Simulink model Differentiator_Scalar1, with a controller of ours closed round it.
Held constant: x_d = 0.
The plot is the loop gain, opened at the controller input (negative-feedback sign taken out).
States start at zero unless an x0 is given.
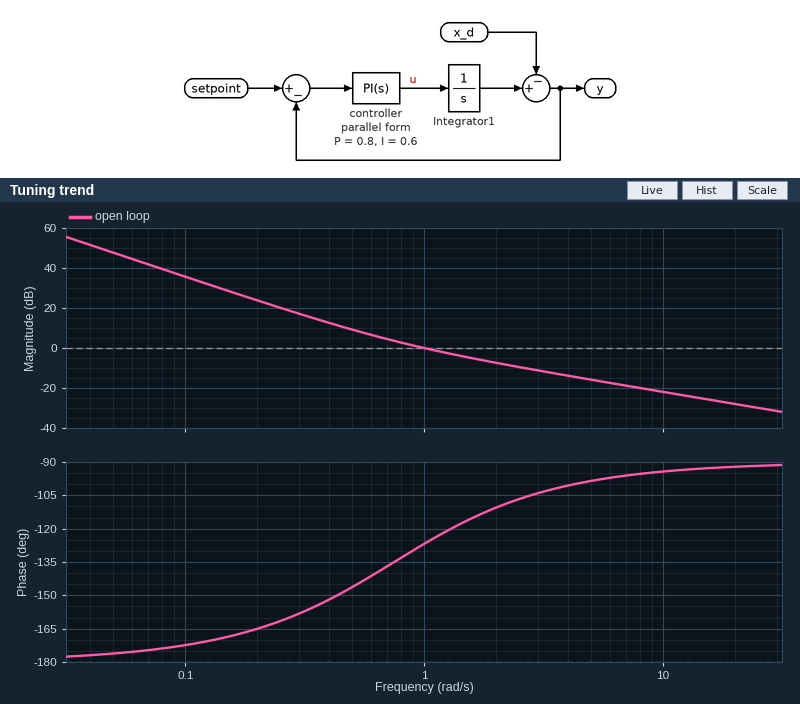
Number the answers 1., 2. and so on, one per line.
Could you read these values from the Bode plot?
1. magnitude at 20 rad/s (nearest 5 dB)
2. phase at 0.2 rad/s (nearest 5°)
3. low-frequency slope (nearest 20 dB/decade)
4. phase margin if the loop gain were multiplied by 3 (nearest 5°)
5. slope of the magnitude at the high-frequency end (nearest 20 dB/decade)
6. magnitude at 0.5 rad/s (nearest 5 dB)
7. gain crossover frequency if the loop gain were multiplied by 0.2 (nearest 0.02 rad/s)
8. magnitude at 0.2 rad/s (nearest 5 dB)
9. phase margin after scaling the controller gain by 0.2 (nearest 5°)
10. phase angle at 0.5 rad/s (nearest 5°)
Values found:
1. -30 dB
2. -165°
3. -40 dB/decade
4. 75°
5. -20 dB/decade
6. 10 dB
7. 0.36 rad/s
8. 25 dB
9. 25°
10. -145°
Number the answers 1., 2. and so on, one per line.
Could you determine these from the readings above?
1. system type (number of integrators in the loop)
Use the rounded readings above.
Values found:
1. 2
